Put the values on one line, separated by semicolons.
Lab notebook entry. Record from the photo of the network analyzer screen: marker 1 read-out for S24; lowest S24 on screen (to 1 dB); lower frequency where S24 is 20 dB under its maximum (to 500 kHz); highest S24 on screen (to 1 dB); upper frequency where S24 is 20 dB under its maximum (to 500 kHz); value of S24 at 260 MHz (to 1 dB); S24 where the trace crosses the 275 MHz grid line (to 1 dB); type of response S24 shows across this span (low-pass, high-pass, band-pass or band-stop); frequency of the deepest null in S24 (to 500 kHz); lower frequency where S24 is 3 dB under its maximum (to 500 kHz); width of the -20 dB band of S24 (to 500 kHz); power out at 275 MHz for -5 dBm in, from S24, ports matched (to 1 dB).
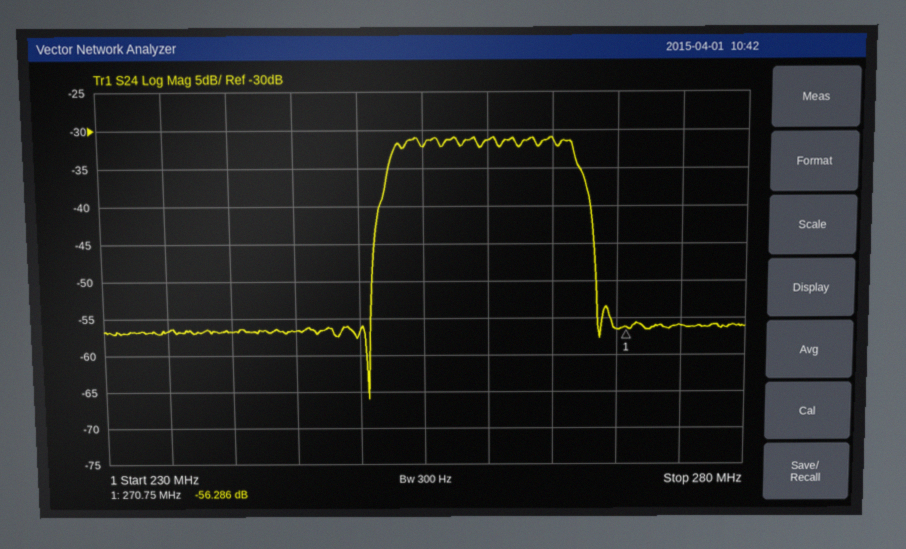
-56.286 dB; -66 dB; 251.0 MHz; -31 dB; 268.5 MHz; -31 dB; -56 dB; band-pass; 250.5 MHz; 252.5 MHz; 17.5 MHz; -61 dBm
